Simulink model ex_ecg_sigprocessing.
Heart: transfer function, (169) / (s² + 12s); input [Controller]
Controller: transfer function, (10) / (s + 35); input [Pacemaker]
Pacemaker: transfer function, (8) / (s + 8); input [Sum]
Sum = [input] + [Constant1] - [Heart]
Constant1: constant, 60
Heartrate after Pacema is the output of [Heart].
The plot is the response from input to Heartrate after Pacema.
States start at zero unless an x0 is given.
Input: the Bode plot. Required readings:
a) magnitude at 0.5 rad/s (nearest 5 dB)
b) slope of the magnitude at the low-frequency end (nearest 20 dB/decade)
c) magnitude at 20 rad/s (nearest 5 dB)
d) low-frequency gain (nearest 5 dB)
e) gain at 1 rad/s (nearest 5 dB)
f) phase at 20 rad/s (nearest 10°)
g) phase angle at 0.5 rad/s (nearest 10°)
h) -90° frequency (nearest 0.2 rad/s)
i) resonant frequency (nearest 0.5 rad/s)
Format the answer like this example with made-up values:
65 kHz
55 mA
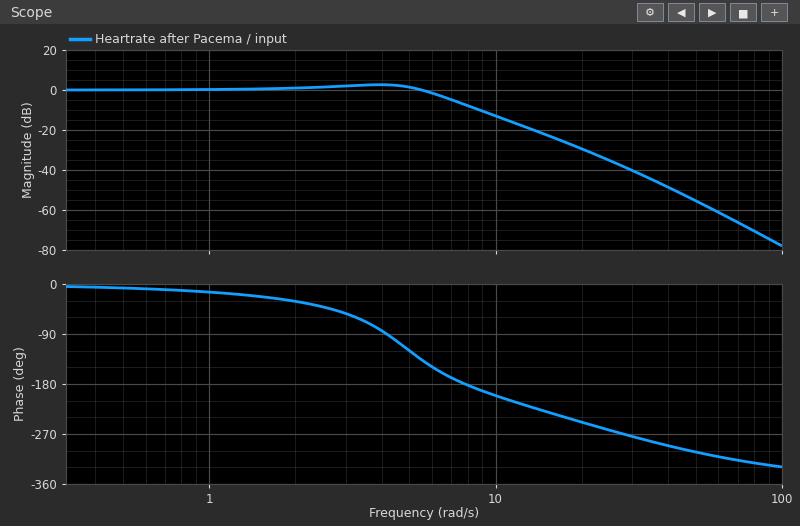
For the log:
0 dB
0 dB/decade
-30 dB
0 dB
0 dB
-250°
-10°
4.2 rad/s
4.0 rad/s
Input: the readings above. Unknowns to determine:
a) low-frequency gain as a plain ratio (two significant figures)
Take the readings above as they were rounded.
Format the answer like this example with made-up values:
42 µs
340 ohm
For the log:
1.0
